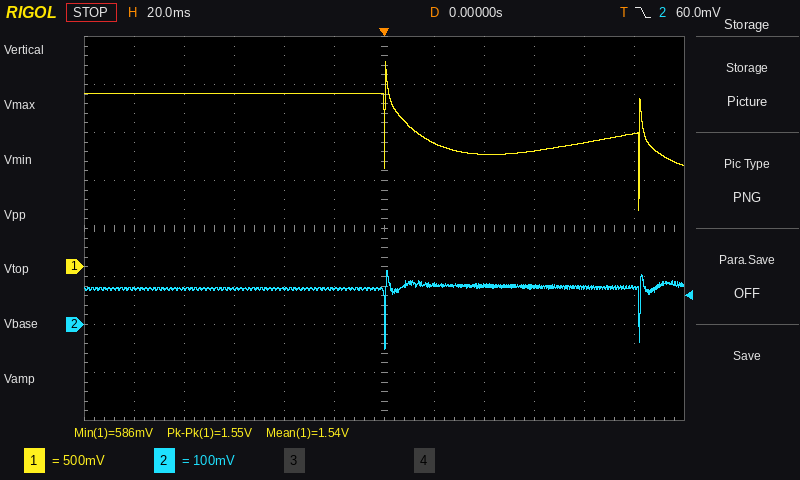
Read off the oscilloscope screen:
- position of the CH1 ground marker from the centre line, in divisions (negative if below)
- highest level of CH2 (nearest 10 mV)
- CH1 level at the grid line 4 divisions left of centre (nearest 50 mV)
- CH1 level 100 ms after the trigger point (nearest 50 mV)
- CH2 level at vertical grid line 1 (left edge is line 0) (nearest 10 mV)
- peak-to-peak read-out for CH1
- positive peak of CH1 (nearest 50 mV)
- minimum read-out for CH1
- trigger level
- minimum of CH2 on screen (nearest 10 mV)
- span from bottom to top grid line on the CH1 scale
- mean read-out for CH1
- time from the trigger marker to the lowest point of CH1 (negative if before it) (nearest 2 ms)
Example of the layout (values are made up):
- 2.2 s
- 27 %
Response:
- -0.8 div
- 110 mV
- 1.80 V
- 1.40 V
- 70 mV
- 1.55 V
- 2.15 V
- 586 mV
- 60.0 mV
- -50 mV
- 4 V
- 1.54 V
- +102 ms
